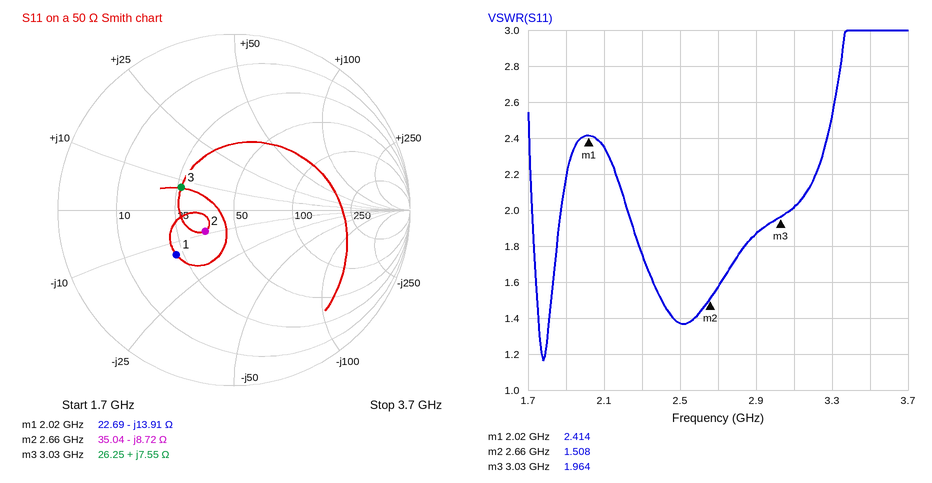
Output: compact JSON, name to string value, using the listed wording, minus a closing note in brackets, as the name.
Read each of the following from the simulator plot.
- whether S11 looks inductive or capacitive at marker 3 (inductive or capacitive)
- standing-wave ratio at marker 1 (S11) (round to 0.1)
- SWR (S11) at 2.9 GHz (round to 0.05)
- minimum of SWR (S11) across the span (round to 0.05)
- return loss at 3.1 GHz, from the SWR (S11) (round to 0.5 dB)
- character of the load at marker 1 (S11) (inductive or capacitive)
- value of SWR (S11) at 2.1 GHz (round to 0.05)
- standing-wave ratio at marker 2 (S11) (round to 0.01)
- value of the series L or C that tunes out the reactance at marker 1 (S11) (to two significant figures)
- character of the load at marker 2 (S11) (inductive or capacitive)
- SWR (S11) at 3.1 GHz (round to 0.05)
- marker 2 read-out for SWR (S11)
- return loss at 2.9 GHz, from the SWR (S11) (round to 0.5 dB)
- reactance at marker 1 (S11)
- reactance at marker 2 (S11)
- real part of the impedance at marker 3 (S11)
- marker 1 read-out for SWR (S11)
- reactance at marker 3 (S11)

{"whether S11 looks inductive or capacitive at marker 3": "inductive", "standing-wave ratio at marker 1 (S11)": "2.4", "SWR (S11) at 2.9 GHz": "1.85", "minimum of SWR (S11) across the span": "1.15", "return loss at 3.1 GHz, from the SWR (S11)": "9.5 dB", "character of the load at marker 1 (S11)": "capacitive", "value of SWR (S11) at 2.1 GHz": "2.35", "standing-wave ratio at marker 2 (S11)": "1.51", "value of the series L or C that tunes out the reactance at marker 1 (S11)": "1.1 nH", "character of the load at marker 2 (S11)": "capacitive", "SWR (S11) at 3.1 GHz": "2.00", "marker 2 read-out for SWR": "1.508", "return loss at 2.9 GHz, from the SWR (S11)": "10.5 dB", "reactance at marker 1": "-13.91 Ω", "reactance at marker 2": "-8.72 Ω", "real part of the impedance at marker 3": "26.25 Ω", "marker 1 read-out for SWR": "2.414", "reactance at marker 3": "+7.55 Ω"}
